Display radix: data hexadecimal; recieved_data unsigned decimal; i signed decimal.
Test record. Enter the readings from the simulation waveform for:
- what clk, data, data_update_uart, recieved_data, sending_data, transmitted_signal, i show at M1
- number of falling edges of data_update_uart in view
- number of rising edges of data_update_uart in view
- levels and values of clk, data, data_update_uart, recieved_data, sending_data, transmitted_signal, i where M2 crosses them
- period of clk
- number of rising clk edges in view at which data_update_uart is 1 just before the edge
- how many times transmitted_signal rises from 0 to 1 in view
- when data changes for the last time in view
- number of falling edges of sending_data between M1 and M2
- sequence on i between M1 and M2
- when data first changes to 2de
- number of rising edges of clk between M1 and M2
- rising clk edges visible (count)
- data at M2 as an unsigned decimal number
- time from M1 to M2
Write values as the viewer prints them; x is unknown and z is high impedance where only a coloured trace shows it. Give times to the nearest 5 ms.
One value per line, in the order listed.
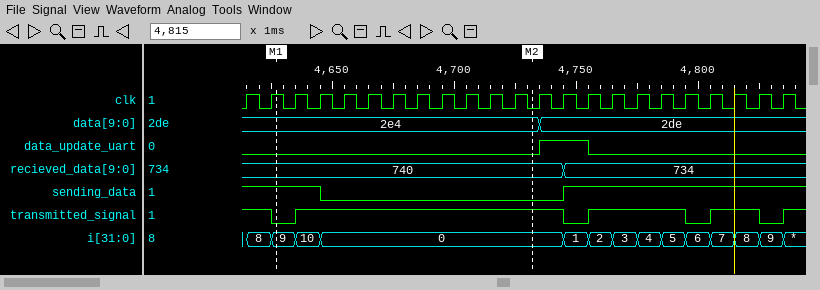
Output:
clk=1, data=2e4, data_update_uart=0, recieved_data=740, sending_data=1, transmitted_signal=0, i=9
1
1
clk=0, data=2e4, data_update_uart=0, recieved_data=740, sending_data=0, transmitted_signal=1, i=0
10 ms
2
4
4735 ms
1
9, 10, 0
4735 ms
10
23
740
105 ms
